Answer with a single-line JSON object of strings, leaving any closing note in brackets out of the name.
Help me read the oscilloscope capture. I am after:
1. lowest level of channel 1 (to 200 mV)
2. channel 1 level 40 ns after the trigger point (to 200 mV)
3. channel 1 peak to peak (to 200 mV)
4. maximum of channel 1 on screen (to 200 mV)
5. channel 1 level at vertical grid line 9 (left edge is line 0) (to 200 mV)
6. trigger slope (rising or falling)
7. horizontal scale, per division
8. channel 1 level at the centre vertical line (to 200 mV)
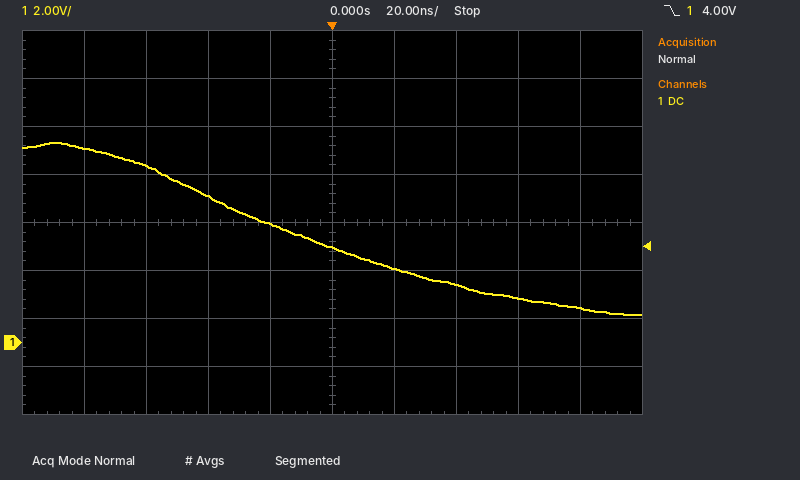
{"lowest level of channel 1": "1.2 V", "channel 1 level 40 ns after the trigger point": "2.4 V", "channel 1 peak to peak": "7.2 V", "maximum of channel 1 on screen": "8.4 V", "channel 1 level at vertical grid line 9 (left edge is line 0)": "1.4 V", "trigger slope": "falling", "horizontal scale, per division": "20 ns", "channel 1 level at the centre vertical line": "4.0 V"}
